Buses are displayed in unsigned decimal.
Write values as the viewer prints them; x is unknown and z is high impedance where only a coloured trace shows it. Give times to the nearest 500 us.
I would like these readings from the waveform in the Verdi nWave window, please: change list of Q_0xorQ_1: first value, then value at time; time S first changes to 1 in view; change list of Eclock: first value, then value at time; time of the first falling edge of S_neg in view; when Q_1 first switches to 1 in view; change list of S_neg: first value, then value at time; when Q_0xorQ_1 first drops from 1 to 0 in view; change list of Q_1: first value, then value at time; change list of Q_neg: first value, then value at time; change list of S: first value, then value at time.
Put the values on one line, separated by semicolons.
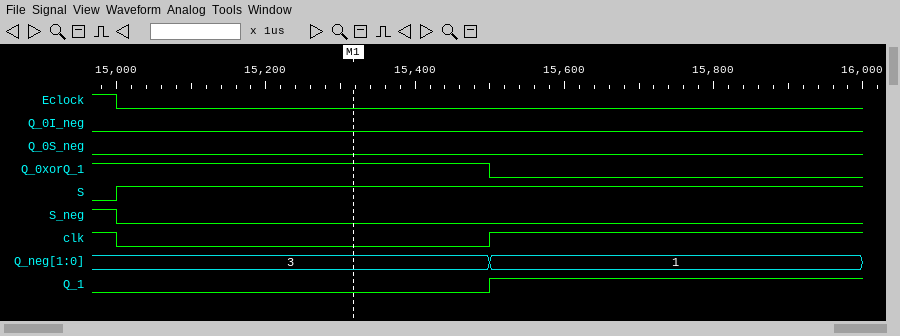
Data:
1, 0 at 15500 us; 15000 us; 1, 0 at 15000 us; 15000 us; 15500 us; 1, 0 at 15000 us; 15500 us; 0, 1 at 15500 us; 3, 1 at 15500 us; 0, 1 at 15000 us
